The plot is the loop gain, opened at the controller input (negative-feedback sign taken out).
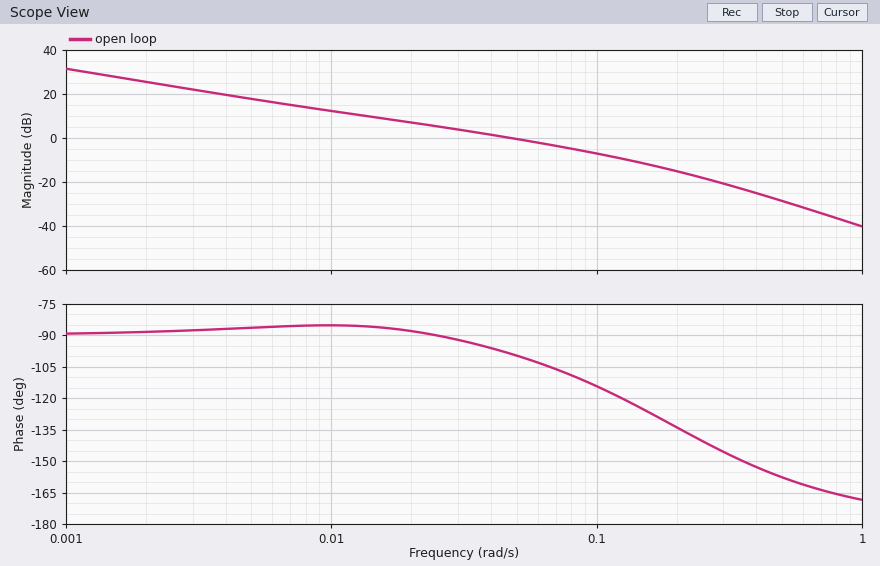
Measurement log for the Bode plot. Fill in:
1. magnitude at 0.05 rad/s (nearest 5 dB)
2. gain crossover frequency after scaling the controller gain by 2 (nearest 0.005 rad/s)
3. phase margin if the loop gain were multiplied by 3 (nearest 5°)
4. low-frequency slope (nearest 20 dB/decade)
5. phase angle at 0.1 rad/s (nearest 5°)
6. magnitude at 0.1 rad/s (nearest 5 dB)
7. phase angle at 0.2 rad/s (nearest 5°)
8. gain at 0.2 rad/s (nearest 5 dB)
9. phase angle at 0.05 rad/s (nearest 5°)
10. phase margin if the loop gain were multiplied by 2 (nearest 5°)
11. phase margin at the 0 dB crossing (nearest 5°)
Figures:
0 dB
0.090 rad/s
60°
-20 dB/decade
-115°
-5 dB
-135°
-15 dB
-100°
70°
80°
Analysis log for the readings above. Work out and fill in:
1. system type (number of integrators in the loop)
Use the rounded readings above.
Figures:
1
